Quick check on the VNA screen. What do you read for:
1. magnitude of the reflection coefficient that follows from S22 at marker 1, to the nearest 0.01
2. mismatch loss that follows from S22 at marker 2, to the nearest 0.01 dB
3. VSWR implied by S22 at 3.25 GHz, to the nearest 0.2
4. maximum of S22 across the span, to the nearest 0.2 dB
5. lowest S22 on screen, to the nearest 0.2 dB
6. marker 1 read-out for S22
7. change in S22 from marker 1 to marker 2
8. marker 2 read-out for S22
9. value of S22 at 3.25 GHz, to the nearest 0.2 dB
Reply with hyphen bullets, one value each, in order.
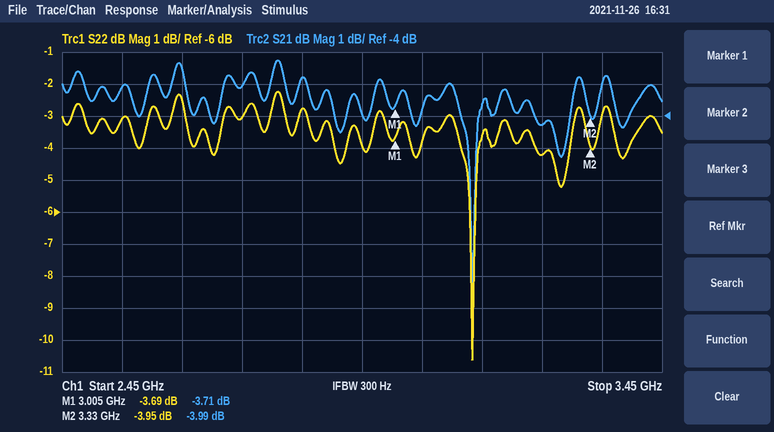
- 0.65
- 2.24 dB
- 4.2
- -2.2 dB
- -10.6 dB
- -3.69 dB
- -0.26 dB
- -3.95 dB
- -4.2 dB
